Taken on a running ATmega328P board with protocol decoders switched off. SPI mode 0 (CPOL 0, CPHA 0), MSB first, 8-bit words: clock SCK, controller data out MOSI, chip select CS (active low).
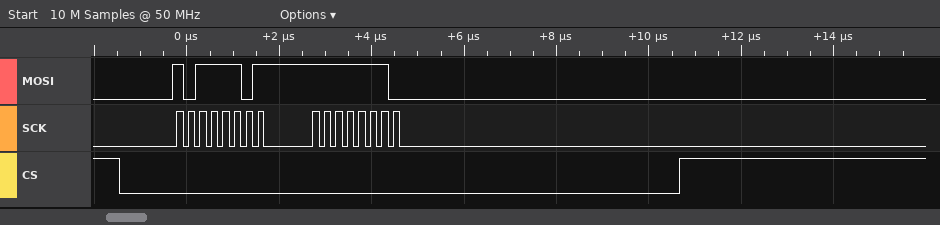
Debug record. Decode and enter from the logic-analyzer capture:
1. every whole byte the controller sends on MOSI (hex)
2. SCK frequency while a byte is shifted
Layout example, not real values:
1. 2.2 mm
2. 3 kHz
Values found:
1. 0xBD 0xFE
2. 4 MHz
